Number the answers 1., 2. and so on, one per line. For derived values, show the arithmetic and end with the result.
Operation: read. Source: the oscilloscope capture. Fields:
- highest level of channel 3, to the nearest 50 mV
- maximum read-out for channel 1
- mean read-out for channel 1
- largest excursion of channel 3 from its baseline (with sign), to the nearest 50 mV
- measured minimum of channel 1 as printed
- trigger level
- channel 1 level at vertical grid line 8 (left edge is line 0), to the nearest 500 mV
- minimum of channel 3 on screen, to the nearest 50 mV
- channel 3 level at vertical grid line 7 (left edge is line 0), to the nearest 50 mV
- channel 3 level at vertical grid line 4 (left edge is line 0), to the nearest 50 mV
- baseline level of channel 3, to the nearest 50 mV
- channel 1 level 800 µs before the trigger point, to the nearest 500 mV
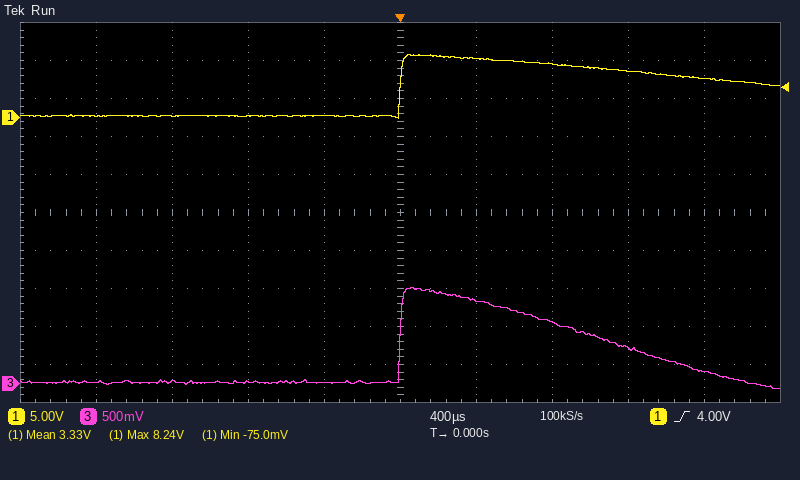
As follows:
1. 1.25 V
2. 8.24 V
3. 3.33 V
4. 1.25 V − (0 mV) = +1.25 V
5. -75.0 mV
6. 4.00 V
7. 6.0 V
8. -50 mV
9. 800 mV
10. 0 mV
11. 0 mV
12. 0.0 V
